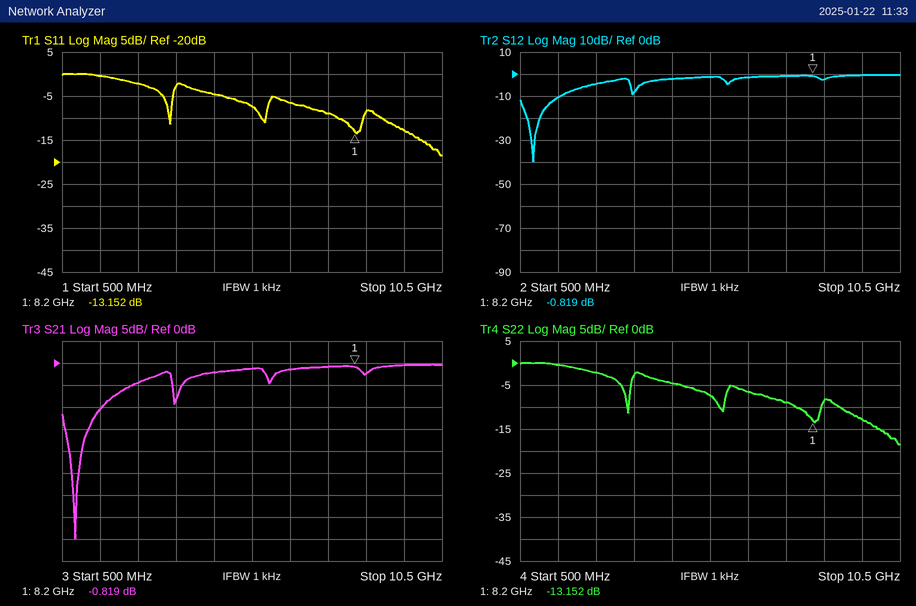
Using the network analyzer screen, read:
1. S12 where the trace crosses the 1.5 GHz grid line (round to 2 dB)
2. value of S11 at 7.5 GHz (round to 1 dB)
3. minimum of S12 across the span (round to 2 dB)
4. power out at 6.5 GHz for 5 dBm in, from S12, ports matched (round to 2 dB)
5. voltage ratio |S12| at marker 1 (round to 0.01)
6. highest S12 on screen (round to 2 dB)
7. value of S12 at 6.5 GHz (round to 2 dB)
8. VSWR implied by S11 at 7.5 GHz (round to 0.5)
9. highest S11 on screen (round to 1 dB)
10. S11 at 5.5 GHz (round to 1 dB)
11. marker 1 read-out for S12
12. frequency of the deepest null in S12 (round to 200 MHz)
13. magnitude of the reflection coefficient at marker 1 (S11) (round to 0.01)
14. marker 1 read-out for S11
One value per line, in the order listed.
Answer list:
-10 dB
-9 dB
-40 dB
4 dBm
0.91
0 dB
-2 dB
2.0
0 dB
-7 dB
-0.819 dB
800 MHz
0.22
-13.152 dB
